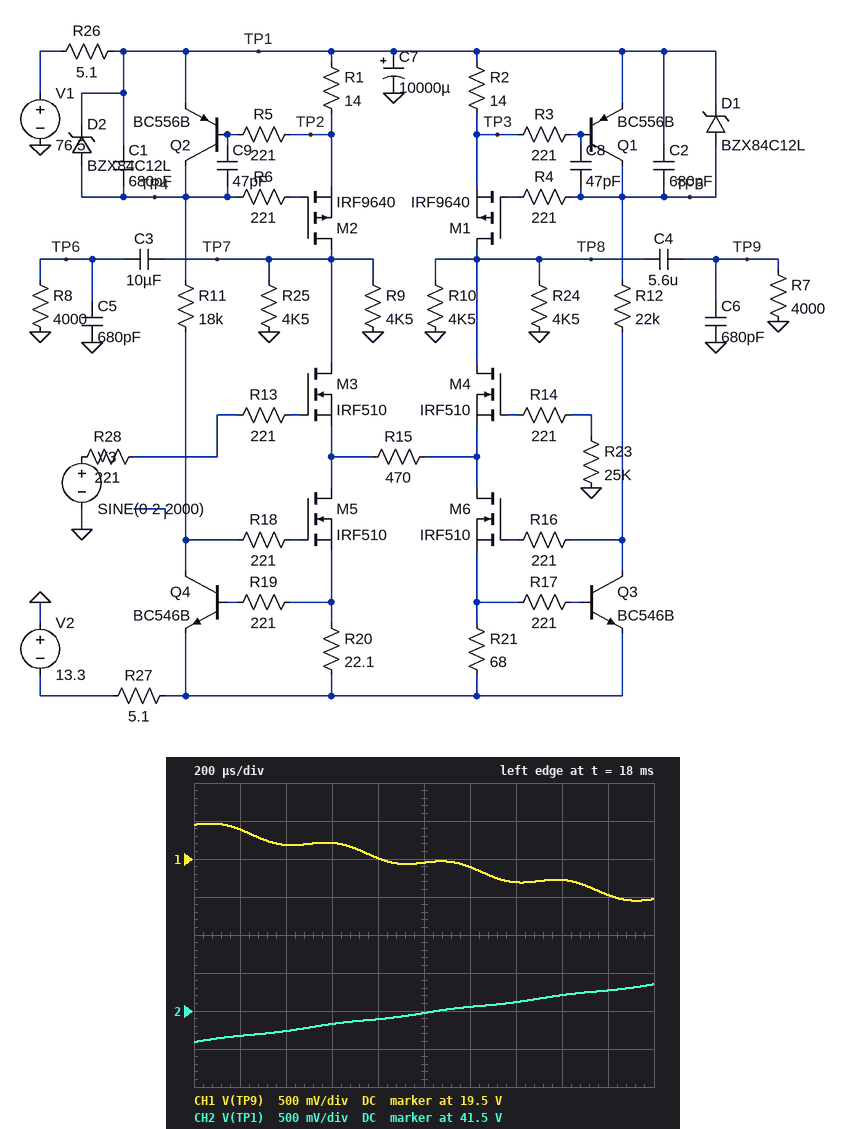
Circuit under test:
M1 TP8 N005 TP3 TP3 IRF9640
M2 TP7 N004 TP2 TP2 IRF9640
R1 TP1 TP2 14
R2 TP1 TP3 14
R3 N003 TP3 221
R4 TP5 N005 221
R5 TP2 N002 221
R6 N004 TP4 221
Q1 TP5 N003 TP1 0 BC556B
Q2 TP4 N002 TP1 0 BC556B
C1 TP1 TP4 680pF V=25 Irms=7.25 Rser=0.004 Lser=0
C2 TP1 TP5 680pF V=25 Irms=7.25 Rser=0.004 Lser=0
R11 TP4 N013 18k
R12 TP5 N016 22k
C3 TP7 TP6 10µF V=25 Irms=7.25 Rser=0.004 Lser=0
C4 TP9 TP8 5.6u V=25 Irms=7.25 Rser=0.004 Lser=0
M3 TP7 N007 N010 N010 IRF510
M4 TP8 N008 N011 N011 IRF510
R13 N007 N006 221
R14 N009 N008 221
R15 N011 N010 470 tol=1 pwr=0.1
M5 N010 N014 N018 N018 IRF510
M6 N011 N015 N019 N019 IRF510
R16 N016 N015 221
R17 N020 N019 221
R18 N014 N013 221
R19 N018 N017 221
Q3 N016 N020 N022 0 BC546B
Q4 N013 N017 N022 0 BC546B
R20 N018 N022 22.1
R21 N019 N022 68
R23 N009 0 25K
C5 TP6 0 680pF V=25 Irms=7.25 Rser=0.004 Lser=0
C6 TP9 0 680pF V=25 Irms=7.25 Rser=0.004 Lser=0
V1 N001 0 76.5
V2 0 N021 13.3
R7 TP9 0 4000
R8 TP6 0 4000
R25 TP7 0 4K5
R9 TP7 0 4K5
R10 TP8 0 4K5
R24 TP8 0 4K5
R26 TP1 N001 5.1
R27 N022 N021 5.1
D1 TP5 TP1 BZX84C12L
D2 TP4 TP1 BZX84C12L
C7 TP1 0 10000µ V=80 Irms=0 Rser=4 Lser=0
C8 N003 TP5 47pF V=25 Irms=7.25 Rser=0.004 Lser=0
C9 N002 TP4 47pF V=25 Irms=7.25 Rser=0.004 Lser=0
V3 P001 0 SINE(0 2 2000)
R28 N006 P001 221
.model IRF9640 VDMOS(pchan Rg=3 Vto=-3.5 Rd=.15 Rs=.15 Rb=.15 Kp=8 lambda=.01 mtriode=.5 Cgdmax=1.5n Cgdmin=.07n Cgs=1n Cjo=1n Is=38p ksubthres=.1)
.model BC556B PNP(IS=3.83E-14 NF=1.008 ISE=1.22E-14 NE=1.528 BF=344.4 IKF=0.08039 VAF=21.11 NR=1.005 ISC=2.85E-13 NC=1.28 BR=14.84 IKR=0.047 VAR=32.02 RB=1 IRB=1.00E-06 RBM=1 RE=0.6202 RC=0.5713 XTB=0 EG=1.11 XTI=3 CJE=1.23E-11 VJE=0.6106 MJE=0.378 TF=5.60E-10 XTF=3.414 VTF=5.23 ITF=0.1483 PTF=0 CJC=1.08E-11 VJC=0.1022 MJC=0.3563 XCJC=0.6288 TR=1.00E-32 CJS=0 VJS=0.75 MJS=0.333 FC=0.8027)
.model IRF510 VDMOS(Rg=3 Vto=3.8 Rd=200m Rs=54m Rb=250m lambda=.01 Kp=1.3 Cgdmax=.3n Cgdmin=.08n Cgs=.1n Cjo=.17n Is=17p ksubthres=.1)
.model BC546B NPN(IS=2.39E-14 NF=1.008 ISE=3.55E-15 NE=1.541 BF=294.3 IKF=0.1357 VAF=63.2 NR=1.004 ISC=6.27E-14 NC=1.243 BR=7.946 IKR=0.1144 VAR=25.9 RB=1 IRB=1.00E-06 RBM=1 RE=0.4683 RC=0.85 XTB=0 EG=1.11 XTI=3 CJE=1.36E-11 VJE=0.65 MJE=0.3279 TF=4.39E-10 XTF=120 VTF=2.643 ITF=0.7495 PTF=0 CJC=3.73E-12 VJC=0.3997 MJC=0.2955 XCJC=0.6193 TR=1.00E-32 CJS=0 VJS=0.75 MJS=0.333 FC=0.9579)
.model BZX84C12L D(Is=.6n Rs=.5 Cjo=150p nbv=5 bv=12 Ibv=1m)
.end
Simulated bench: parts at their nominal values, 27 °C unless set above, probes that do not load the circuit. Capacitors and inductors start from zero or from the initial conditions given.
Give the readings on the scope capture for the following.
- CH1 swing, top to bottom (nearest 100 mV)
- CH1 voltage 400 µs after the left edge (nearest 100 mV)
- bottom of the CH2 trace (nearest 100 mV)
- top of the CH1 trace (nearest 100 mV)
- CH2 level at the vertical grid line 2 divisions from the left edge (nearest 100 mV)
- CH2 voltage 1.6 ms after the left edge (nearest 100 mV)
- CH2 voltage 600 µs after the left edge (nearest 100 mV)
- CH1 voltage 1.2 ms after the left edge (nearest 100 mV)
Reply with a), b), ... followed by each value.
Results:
a) 1.0 V
b) 19.7 V
c) 41.1 V
d) 20.0 V
e) 41.2 V
f) 41.7 V
g) 41.3 V
h) 19.4 V
